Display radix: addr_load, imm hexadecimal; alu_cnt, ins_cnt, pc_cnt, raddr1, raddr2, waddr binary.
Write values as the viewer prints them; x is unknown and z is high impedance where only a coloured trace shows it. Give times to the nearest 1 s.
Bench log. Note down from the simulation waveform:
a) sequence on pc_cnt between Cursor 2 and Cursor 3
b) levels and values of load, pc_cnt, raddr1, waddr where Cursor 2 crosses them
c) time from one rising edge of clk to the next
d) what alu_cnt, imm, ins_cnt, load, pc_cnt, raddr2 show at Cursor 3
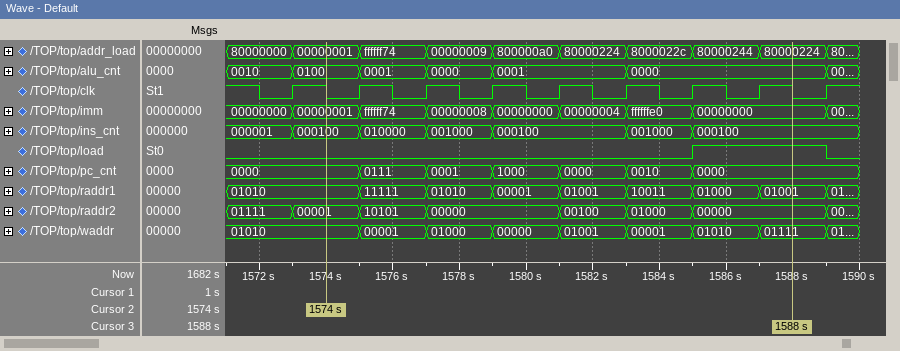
0000, 0111, 0001, 1000, 0000, 0010, 0000
load=0, pc_cnt=0000, raddr1=01010, waddr=01010
2 s
alu_cnt=0000, imm=00000000, ins_cnt=000100, load=1, pc_cnt=0000, raddr2=00000
